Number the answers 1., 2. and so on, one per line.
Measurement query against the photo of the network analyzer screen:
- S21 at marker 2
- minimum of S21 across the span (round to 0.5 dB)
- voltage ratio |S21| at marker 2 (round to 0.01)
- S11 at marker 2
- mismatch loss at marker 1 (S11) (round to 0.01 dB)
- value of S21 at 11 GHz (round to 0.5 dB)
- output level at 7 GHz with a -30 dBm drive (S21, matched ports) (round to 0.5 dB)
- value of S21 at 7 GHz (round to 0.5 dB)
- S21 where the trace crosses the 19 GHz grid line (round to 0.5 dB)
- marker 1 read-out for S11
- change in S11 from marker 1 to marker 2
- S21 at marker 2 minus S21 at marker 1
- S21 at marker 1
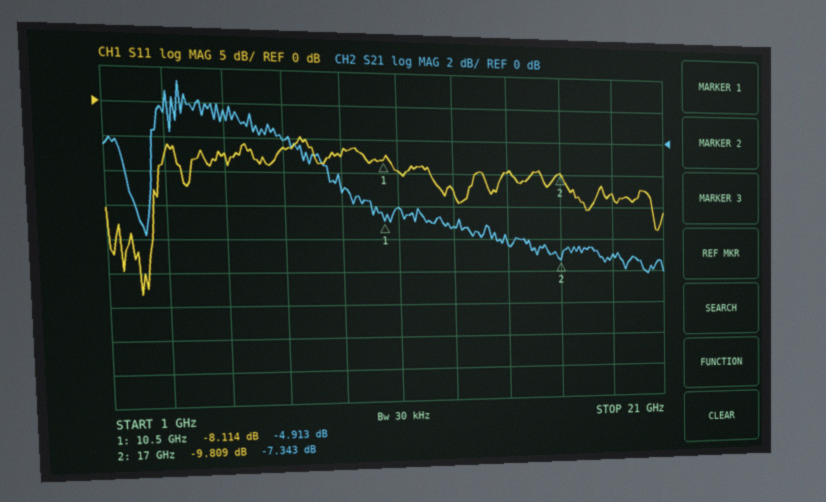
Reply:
1. -7.343 dB
2. -8.0 dB
3. 0.43
4. -9.809 dB
5. 0.73 dB
6. -4.0 dB
7. -30.0 dBm
8. 0.0 dB
9. -7.0 dB
10. -8.114 dB
11. -1.695 dB
12. -2.430 dB
13. -4.913 dB
